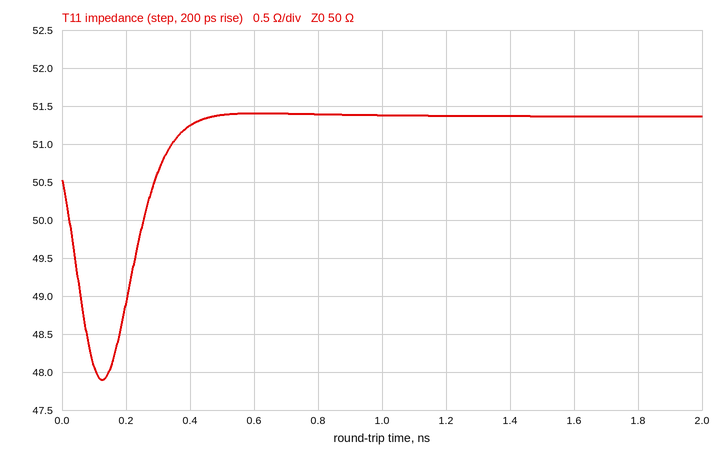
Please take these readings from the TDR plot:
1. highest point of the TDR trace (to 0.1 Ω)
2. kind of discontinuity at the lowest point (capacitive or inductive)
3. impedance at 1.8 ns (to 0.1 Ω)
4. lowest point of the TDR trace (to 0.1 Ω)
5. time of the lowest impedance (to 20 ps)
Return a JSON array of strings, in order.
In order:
["51.4 Ω", "capacitive", "51.4 Ω", "47.9 Ω", "120 ps"]
